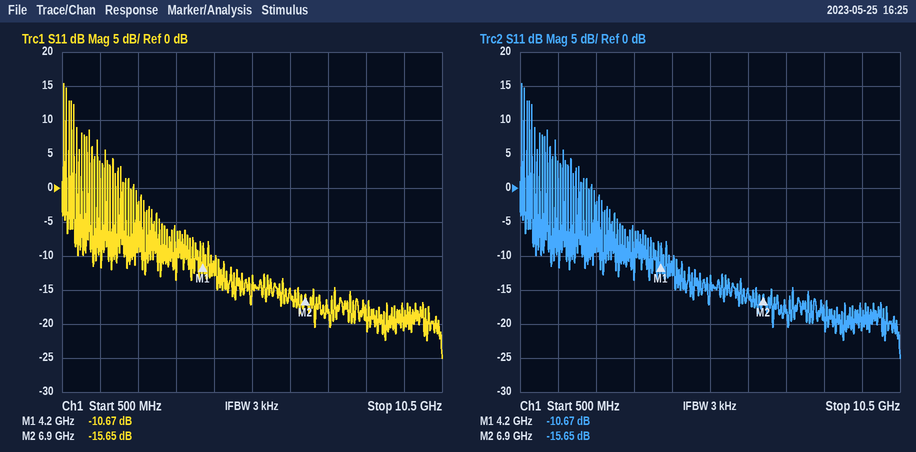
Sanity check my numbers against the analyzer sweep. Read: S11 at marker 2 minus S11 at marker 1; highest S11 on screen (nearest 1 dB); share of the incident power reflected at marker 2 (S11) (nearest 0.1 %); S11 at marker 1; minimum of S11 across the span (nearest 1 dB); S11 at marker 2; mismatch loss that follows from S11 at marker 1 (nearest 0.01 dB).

-4.98 dB
15 dB
2.7 %
-10.67 dB
-25 dB
-15.65 dB
0.39 dB
